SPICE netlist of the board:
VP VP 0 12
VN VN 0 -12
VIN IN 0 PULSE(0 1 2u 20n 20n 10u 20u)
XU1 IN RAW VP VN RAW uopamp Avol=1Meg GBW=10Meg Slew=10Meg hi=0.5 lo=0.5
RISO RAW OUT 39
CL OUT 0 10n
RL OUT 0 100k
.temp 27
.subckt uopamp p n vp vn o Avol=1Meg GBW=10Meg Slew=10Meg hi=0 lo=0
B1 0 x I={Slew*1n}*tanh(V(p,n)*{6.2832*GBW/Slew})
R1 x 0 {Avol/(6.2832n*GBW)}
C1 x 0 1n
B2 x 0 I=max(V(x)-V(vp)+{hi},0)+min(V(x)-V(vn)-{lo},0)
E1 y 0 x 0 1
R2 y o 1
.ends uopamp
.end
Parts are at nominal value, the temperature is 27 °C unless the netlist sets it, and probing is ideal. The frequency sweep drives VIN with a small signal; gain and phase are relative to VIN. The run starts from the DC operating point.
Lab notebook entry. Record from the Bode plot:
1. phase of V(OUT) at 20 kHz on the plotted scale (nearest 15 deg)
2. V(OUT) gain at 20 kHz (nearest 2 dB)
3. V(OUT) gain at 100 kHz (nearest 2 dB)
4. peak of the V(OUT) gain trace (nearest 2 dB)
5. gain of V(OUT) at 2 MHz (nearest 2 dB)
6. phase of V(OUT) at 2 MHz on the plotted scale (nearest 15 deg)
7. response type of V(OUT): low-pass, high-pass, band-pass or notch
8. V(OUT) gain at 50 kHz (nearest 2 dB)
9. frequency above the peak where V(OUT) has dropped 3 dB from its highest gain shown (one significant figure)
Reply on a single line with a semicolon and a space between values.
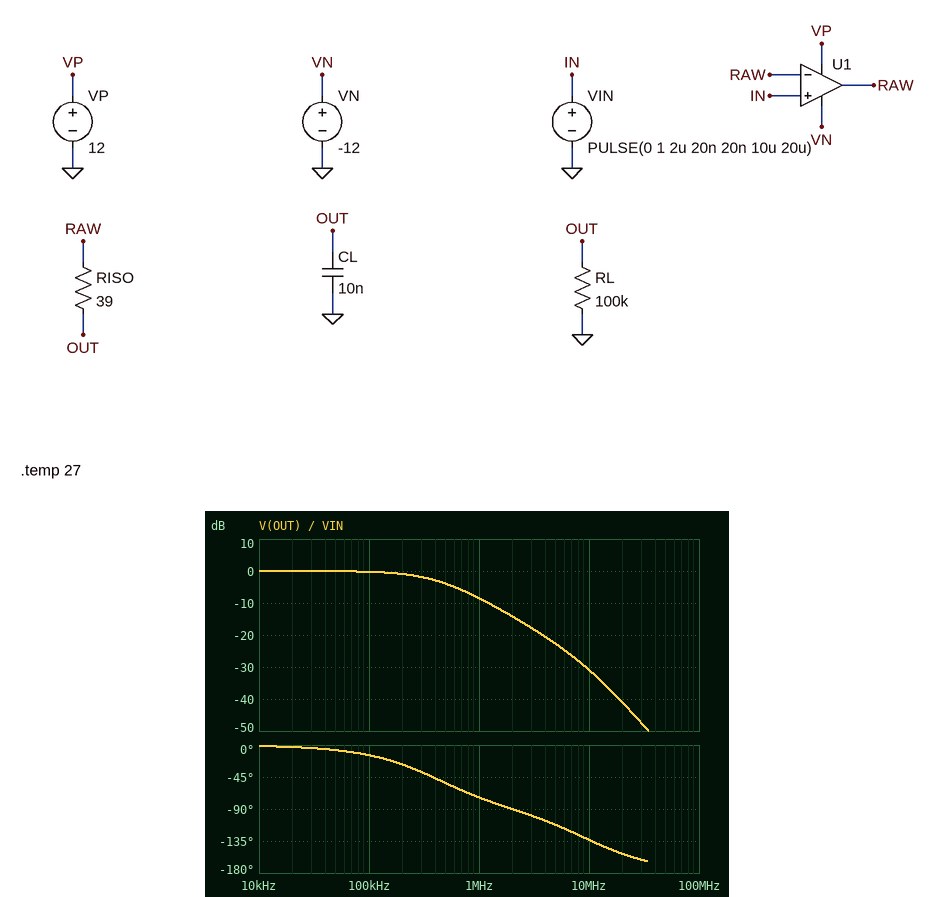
0 deg; 0 dB; 0 dB; 0 dB; -14 dB; -90 deg; low-pass; 0 dB; 400 kHz
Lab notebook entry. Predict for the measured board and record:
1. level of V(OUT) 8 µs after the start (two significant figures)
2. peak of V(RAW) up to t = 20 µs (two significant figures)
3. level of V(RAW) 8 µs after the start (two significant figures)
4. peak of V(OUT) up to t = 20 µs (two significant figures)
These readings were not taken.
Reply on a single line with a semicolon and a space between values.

1.0 V; 1.0 V; 1.0 V; 1.0 V
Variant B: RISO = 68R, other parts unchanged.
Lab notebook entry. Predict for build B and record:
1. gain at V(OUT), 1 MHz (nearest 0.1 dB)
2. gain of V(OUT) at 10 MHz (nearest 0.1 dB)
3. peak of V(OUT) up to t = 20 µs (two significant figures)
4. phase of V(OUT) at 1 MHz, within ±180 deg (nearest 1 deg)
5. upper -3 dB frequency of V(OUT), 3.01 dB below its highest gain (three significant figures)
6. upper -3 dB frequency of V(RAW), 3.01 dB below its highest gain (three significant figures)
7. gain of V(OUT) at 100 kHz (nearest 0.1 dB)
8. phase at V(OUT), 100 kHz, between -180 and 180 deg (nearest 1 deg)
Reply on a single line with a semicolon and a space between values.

-12.9 dB; -35.7 dB; 1.0 V; -83 deg; 234 kHz; 9.86 MHz; -0.7 dB; -24 deg
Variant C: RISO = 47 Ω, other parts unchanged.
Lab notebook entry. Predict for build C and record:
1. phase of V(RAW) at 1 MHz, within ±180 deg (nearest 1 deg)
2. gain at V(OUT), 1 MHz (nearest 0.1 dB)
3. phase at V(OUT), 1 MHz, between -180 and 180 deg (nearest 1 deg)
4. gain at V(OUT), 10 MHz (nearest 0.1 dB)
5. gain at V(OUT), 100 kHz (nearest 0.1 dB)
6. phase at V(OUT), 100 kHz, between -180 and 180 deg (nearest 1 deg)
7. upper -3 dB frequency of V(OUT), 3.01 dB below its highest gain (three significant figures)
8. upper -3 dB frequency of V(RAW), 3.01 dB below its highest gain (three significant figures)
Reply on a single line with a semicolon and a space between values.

-6 deg; -9.9 dB; -77 deg; -32.5 dB; -0.4 dB; -17 deg; 339 kHz; 9.80 MHz
